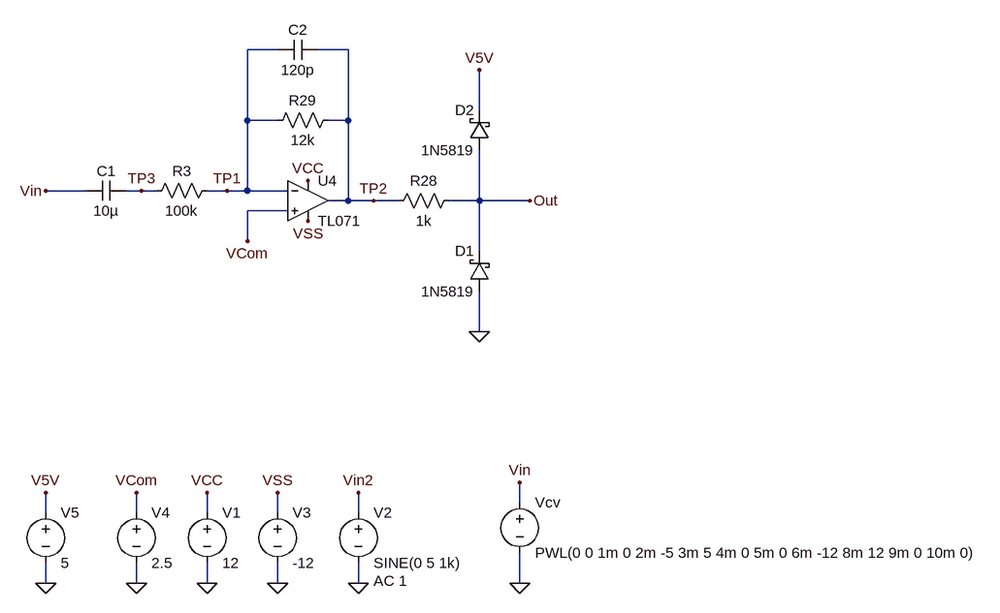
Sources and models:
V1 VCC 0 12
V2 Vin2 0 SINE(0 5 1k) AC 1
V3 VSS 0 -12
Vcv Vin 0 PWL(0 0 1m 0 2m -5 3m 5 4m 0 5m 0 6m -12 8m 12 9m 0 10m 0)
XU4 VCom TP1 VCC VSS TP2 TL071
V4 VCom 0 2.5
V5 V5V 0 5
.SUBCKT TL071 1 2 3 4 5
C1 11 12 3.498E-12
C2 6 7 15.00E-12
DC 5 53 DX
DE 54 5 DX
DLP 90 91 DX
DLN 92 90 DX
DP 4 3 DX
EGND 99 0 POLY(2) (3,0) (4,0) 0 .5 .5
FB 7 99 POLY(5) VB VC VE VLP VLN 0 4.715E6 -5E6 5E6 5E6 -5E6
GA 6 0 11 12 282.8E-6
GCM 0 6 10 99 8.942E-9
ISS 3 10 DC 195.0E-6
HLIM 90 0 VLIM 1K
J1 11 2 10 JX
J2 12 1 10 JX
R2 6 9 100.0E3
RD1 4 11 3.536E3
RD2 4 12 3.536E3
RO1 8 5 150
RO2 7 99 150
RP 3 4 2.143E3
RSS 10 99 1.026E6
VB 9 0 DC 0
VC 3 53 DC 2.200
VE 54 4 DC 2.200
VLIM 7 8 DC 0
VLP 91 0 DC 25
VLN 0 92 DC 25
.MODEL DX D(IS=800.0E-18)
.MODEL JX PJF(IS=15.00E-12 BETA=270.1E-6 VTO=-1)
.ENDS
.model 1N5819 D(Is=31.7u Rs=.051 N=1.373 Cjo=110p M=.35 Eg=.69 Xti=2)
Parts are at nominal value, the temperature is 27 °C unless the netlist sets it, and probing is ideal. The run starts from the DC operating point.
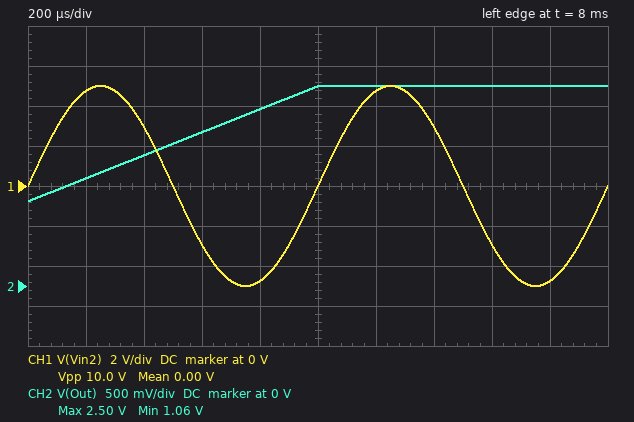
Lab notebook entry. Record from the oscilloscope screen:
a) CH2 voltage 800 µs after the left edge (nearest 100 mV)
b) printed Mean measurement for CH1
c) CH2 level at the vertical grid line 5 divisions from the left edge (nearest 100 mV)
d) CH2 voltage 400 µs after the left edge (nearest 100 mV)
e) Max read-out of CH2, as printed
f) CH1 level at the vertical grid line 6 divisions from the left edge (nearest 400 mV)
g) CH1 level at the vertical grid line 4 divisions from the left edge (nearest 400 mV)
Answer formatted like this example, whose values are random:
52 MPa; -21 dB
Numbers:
2.2 V; 0.00 V; 2.5 V; 1.6 V; 2.50 V; 4.8 V; -4.8 V
